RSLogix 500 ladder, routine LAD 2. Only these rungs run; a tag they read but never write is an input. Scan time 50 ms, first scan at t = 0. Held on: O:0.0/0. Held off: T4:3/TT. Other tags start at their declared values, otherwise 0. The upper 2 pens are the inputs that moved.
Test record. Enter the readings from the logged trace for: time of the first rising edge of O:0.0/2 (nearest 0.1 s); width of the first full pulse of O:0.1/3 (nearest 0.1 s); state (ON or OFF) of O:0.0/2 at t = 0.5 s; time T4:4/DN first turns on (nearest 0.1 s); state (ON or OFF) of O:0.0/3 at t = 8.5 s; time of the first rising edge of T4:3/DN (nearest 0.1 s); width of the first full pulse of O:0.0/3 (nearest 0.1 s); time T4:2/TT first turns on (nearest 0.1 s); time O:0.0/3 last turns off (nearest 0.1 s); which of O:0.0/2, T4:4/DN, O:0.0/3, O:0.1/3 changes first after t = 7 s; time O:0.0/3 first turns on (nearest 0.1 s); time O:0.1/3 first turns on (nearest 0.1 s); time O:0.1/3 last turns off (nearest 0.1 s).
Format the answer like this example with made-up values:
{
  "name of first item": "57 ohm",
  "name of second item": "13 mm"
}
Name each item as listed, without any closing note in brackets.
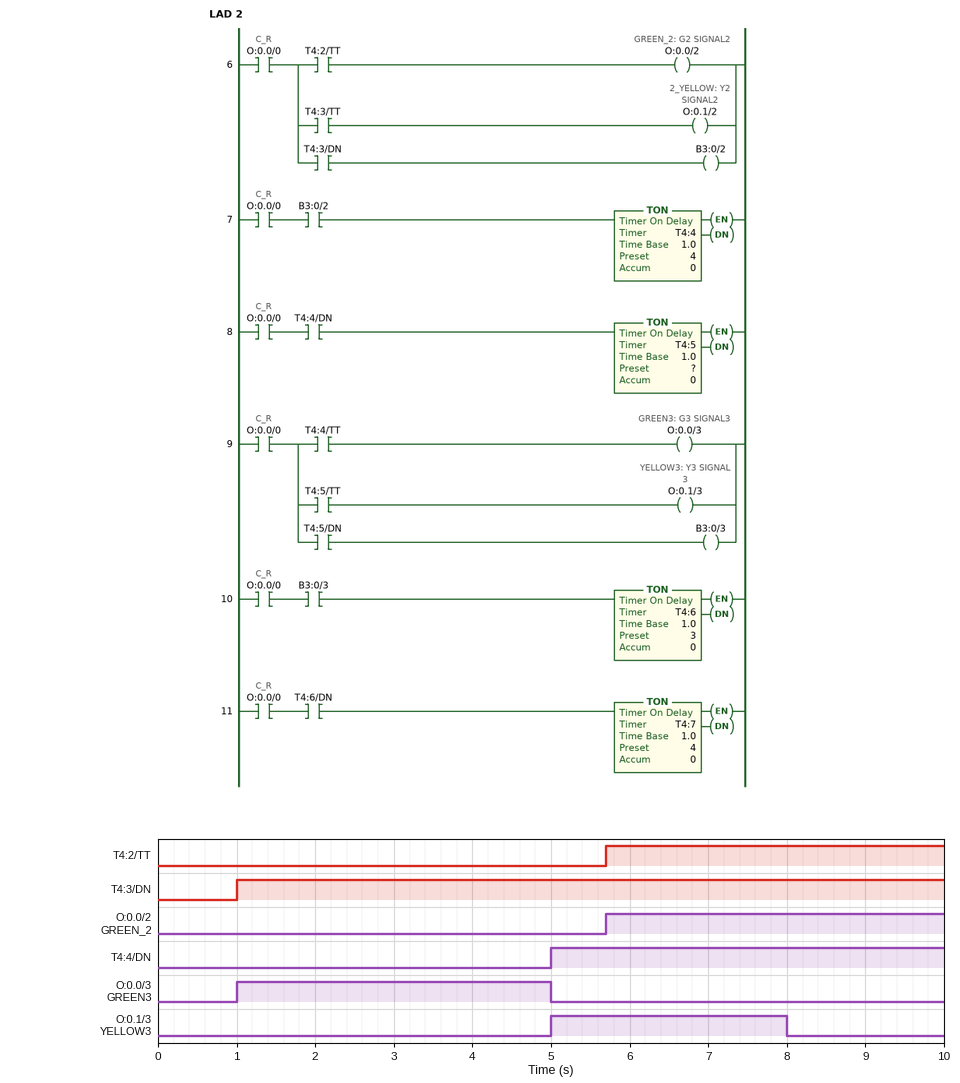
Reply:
{
  "time of the first rising edge of O:0.0/2": "5.7 s",
  "width of the first full pulse of O:0.1/3": "3.0 s",
  "state (ON or OFF) of O:0.0/2 at t = 0.5 s": "OFF",
  "time T4:4/DN first turns on": "5.0 s",
  "state (ON or OFF) of O:0.0/3 at t = 8.5 s": "OFF",
  "time of the first rising edge of T4:3/DN": "1.0 s",
  "width of the first full pulse of O:0.0/3": "4.0 s",
  "time T4:2/TT first turns on": "5.7 s",
  "time O:0.0/3 last turns off": "5.0 s",
  "which of O:0.0/2, T4:4/DN, O:0.0/3, O:0.1/3 changes first after t = 7 s": "O:0.1/3",
  "time O:0.0/3 first turns on": "1.0 s",
  "time O:0.1/3 first turns on": "5.0 s",
  "time O:0.1/3 last turns off": "8.0 s"
}
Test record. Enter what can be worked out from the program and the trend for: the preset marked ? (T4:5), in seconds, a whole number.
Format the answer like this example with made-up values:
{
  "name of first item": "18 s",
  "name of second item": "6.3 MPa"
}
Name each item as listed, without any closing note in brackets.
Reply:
{
  "the preset marked ? (T4:5), in seconds, a whole number": "3 s"
}
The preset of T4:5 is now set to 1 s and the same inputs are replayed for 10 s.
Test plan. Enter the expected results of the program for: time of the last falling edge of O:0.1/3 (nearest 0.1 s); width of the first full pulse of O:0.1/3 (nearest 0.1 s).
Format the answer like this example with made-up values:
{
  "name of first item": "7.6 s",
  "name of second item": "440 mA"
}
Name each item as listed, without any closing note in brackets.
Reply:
{
  "time of the last falling edge of O:0.1/3": "6.0 s",
  "width of the first full pulse of O:0.1/3": "1.0 s"
}
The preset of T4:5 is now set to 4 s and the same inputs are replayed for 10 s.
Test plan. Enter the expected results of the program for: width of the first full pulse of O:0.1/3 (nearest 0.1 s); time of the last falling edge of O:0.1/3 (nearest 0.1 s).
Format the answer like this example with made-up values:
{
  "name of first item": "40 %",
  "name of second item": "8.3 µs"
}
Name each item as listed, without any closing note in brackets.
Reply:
{
  "width of the first full pulse of O:0.1/3": "4.0 s",
  "time of the last falling edge of O:0.1/3": "9.0 s"
}
